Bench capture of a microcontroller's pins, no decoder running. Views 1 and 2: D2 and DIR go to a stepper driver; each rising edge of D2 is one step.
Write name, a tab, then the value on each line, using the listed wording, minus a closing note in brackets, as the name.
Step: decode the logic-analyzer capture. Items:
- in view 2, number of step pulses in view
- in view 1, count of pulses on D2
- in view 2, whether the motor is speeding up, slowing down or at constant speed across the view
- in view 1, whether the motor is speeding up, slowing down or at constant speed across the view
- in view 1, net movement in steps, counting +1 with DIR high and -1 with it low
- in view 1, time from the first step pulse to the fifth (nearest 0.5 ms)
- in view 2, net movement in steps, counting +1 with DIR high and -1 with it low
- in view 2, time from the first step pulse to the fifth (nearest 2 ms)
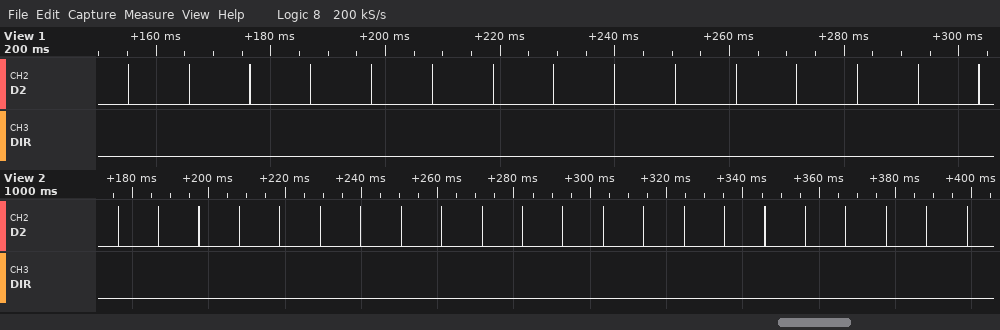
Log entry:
in view 2, number of step pulses in view	22
in view 1, count of pulses on D2	15
in view 2, whether the motor is speeding up, slowing down or at constant speed across the view	constant speed
in view 1, whether the motor is speeding up, slowing down or at constant speed across the view	constant speed
in view 1, net movement in steps, counting +1 with DIR high and -1 with it low	-15
in view 1, time from the first step pulse to the fifth	42.5 ms
in view 2, net movement in steps, counting +1 with DIR high and -1 with it low	-22
in view 2, time from the first step pulse to the fifth	42 ms
